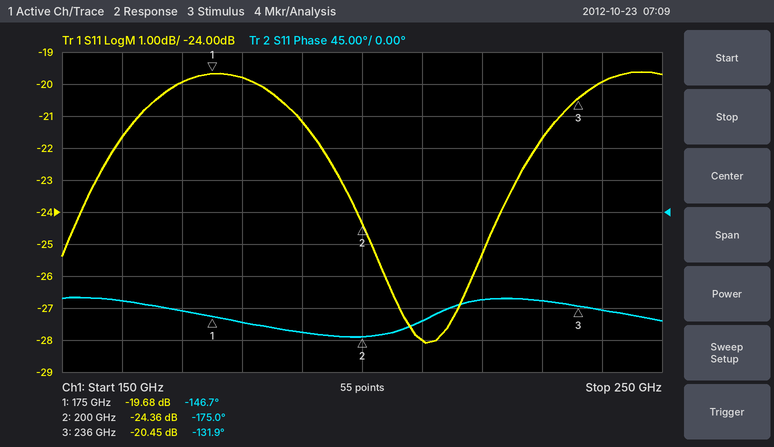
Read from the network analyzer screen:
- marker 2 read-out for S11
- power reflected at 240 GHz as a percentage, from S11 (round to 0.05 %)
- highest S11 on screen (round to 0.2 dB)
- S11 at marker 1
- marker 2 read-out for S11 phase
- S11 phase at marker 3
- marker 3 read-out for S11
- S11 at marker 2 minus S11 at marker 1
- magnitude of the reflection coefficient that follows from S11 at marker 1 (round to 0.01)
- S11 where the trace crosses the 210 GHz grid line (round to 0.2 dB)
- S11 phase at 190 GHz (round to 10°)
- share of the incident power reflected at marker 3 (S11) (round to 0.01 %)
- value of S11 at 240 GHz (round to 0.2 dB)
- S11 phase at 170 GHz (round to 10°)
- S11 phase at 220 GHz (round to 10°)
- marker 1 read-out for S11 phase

-24.36 dB
1.00 %
-19.6 dB
-19.68 dB
-175.0°
-131.9°
-20.45 dB
-4.68 dB
0.10
-28.0 dB
-170°
0.90 %
-20.0 dB
-140°
-120°
-146.7°
